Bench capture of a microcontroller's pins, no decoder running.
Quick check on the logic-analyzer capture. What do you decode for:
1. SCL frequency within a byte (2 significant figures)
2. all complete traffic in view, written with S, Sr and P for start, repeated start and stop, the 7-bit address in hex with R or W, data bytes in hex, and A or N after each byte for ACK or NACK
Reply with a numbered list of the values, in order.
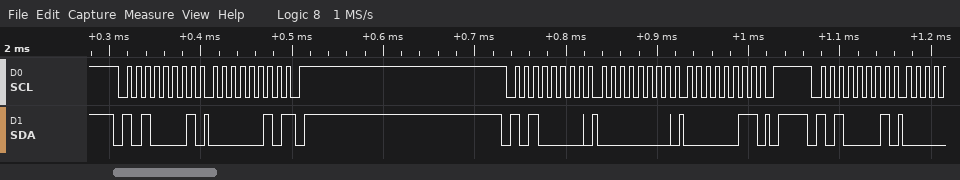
1. 100 kHz
2. S 50R A 02 N P S 50W A 00 A 03 A P S 50R A
